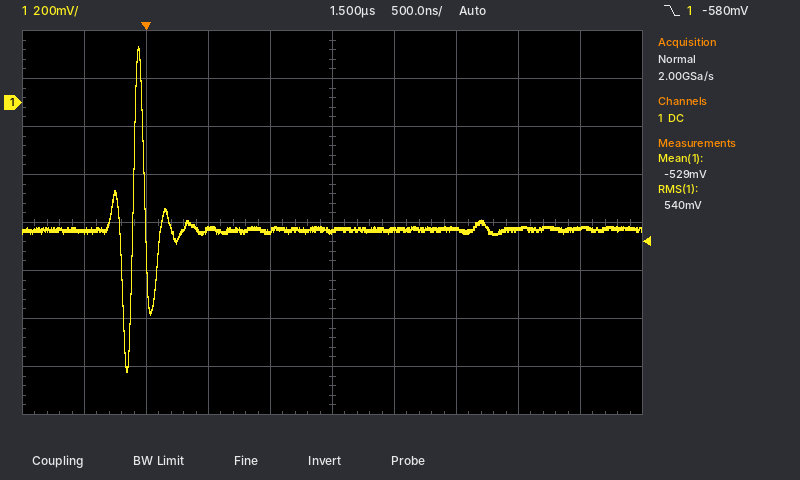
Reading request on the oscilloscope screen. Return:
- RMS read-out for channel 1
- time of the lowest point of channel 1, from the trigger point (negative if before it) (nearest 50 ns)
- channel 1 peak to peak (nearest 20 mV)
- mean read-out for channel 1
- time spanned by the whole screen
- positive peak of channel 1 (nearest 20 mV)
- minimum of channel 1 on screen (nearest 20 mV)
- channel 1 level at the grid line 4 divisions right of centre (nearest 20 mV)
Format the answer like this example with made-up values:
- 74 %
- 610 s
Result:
- 540 mV
- -150 ns
- 1.36 V
- -529 mV
- 5 µs
- 240 mV
- -1.12 V
- -520 mV
